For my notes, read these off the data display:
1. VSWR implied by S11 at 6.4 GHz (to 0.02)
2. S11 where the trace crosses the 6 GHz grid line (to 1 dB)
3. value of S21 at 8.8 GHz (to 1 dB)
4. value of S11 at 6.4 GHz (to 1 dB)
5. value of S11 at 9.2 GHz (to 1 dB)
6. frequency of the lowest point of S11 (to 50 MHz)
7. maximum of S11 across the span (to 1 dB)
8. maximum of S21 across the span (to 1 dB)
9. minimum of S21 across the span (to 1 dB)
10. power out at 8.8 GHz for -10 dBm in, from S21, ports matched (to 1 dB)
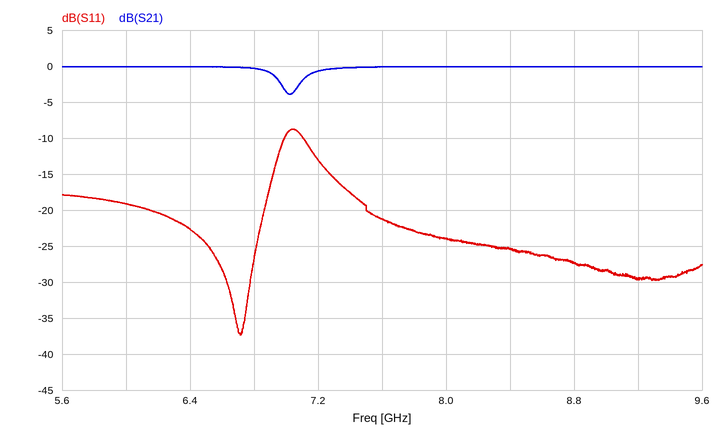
1.16
-19 dB
0 dB
-23 dB
-30 dB
6.70 GHz
-9 dB
0 dB
-4 dB
-10 dBm
